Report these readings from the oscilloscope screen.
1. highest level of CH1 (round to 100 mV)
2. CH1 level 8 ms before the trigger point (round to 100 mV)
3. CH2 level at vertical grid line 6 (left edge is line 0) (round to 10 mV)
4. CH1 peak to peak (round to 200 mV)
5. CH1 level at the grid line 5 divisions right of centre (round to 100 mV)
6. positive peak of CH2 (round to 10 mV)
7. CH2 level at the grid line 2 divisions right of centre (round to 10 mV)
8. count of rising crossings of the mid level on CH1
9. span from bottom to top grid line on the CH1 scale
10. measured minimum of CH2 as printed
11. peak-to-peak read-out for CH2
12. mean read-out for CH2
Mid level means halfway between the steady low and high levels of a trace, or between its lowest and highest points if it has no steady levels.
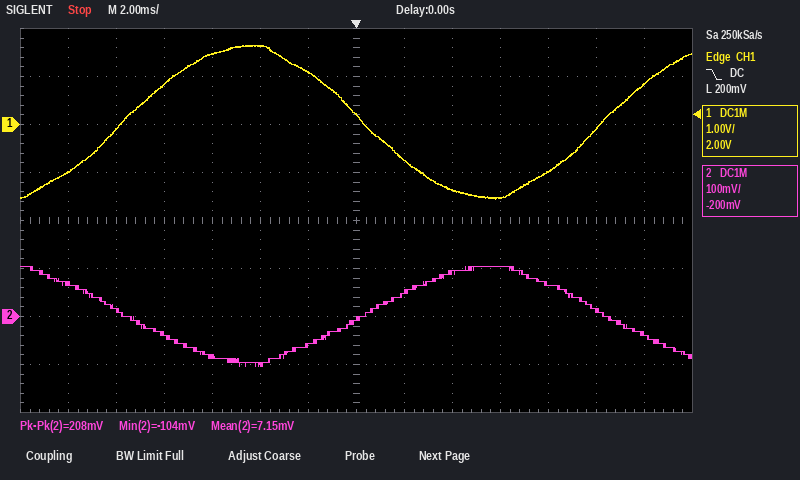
1.6 V
800 mV
-60 mV
3.2 V
-100 mV
100 mV
90 mV
2
8 V
-104 mV
208 mV
7.15 mV
